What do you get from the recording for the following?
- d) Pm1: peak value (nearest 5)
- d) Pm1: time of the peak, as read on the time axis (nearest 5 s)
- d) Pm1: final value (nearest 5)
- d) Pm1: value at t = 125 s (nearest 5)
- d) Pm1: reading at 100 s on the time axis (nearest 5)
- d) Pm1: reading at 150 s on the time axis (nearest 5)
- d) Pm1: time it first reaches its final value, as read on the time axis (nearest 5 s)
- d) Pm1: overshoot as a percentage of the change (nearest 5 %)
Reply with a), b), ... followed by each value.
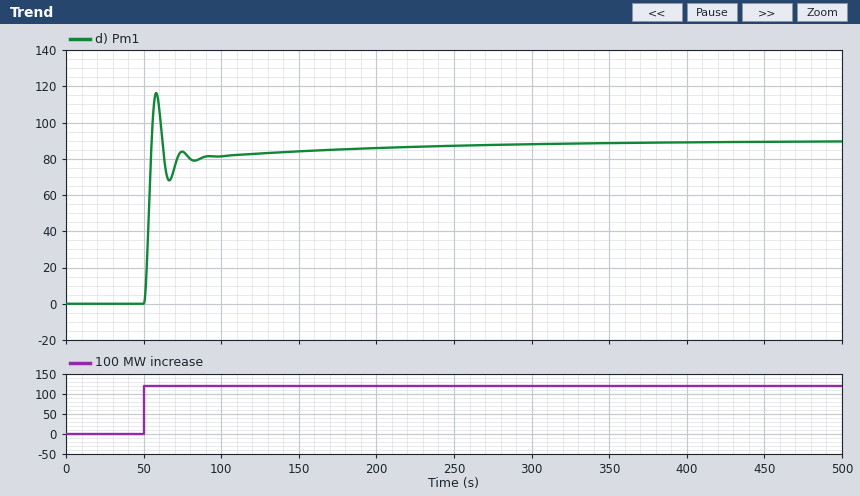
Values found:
a) 115
b) 60 s
c) 90
d) 85
e) 80
f) 85
g) 55 s
h) 30 %
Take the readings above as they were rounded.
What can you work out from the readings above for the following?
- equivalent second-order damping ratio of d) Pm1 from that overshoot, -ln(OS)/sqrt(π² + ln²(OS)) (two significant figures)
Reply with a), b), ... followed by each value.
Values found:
a) 0.36
